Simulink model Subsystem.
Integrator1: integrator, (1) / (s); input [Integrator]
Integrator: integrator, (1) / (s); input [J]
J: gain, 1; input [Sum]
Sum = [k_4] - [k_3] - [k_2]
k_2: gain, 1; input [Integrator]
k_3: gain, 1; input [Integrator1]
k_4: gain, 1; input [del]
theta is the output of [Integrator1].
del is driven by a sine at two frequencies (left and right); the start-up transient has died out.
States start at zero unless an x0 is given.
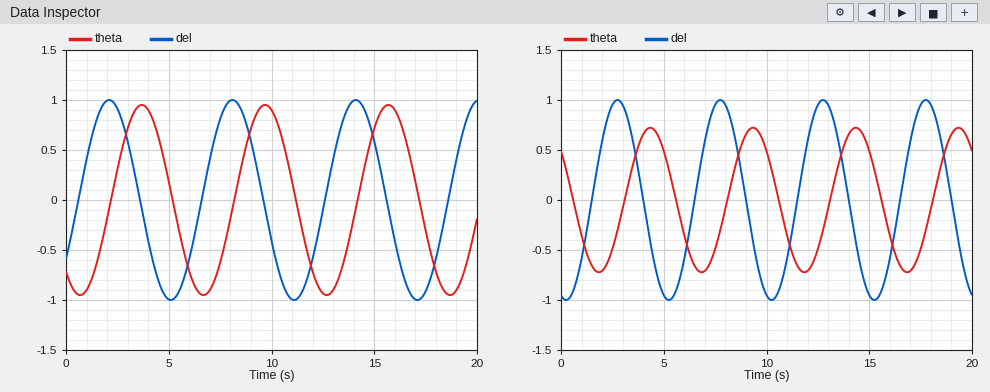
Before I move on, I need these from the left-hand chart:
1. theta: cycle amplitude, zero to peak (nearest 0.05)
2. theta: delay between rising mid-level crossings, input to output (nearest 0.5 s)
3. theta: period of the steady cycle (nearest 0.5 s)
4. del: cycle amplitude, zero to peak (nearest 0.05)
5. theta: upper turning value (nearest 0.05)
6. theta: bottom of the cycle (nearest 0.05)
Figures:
0.95
1.5 s
6.0 s
1.00
0.95
-0.95
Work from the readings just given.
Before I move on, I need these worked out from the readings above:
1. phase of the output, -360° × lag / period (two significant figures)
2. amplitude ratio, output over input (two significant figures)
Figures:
-90°
0.95
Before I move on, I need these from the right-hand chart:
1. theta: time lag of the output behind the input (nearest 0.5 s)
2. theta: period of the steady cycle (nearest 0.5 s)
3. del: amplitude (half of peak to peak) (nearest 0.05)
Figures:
1.5 s
5.0 s
1.00
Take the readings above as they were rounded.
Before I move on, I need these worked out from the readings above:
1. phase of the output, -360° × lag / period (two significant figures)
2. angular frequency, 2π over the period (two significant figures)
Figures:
-110°
1.3 rad/s
